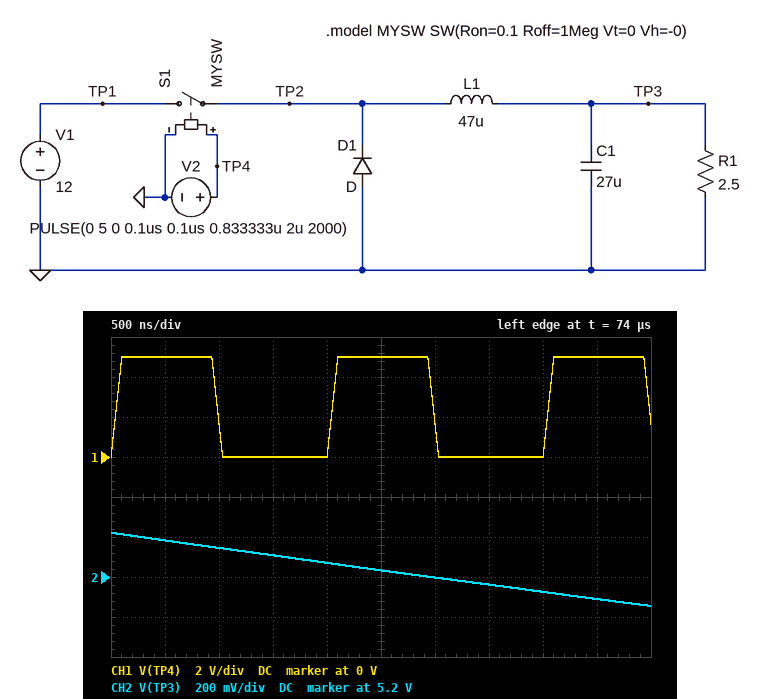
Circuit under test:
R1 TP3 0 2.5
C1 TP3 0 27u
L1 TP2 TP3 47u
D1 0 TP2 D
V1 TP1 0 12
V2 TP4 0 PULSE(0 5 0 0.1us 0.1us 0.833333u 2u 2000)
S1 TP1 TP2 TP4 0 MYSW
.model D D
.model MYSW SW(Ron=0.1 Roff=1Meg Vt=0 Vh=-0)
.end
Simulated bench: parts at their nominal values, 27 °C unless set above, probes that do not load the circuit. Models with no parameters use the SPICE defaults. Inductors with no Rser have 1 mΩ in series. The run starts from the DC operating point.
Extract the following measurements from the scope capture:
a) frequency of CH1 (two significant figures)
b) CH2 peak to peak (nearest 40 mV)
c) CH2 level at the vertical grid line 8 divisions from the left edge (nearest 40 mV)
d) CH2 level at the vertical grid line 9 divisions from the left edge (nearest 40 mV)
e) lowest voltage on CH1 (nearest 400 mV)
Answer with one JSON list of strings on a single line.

["500 kHz", "360 mV", "5.12 V", "5.08 V", "0 V"]
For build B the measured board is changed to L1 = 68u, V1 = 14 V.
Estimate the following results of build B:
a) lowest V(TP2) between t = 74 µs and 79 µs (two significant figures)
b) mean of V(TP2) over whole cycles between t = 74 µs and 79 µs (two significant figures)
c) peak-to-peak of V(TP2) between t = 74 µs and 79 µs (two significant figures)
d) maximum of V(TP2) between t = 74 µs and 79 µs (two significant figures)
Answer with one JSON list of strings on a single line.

["-820 mV", "6.8 V", "15 V", "14 V"]
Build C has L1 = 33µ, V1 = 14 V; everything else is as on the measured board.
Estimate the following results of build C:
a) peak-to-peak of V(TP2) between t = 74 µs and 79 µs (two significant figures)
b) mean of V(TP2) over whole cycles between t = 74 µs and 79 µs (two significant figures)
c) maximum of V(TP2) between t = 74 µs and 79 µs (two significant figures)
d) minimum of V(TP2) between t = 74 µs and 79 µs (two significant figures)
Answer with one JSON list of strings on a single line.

["15 V", "6.8 V", "14 V", "-820 mV"]
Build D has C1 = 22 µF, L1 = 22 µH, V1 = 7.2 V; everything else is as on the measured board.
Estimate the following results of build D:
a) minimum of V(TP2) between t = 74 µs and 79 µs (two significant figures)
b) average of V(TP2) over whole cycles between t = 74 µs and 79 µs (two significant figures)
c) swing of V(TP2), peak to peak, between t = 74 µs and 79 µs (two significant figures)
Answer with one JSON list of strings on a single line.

["-830 mV", "3.3 V", "8.0 V"]
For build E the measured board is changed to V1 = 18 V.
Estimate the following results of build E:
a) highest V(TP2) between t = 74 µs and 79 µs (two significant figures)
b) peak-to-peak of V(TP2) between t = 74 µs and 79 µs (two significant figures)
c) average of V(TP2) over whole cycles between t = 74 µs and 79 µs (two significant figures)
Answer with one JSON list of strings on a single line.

["18 V", "19 V", "8.9 V"]
